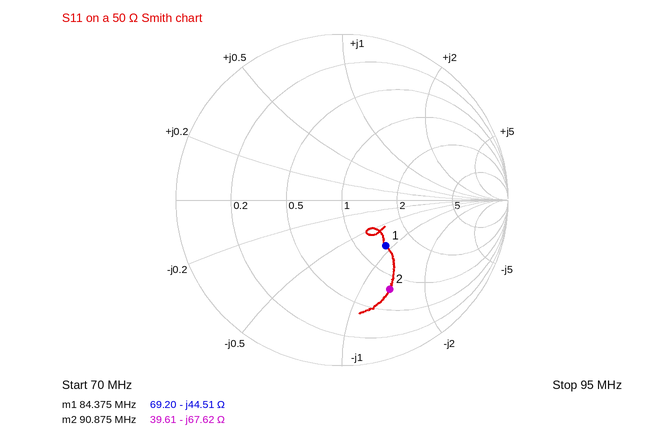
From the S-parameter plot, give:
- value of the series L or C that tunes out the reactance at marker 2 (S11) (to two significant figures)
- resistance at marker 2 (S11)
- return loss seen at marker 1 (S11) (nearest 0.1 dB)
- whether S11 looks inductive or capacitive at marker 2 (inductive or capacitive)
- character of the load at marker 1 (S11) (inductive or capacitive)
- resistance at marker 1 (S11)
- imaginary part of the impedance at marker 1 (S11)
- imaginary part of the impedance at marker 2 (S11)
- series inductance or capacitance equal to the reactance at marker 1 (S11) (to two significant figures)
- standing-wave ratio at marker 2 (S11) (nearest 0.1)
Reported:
120 nH
39.61 Ω
8.4 dB
capacitive
capacitive
69.20 Ω
-44.51 Ω
-67.62 Ω
42 pF
4.1
